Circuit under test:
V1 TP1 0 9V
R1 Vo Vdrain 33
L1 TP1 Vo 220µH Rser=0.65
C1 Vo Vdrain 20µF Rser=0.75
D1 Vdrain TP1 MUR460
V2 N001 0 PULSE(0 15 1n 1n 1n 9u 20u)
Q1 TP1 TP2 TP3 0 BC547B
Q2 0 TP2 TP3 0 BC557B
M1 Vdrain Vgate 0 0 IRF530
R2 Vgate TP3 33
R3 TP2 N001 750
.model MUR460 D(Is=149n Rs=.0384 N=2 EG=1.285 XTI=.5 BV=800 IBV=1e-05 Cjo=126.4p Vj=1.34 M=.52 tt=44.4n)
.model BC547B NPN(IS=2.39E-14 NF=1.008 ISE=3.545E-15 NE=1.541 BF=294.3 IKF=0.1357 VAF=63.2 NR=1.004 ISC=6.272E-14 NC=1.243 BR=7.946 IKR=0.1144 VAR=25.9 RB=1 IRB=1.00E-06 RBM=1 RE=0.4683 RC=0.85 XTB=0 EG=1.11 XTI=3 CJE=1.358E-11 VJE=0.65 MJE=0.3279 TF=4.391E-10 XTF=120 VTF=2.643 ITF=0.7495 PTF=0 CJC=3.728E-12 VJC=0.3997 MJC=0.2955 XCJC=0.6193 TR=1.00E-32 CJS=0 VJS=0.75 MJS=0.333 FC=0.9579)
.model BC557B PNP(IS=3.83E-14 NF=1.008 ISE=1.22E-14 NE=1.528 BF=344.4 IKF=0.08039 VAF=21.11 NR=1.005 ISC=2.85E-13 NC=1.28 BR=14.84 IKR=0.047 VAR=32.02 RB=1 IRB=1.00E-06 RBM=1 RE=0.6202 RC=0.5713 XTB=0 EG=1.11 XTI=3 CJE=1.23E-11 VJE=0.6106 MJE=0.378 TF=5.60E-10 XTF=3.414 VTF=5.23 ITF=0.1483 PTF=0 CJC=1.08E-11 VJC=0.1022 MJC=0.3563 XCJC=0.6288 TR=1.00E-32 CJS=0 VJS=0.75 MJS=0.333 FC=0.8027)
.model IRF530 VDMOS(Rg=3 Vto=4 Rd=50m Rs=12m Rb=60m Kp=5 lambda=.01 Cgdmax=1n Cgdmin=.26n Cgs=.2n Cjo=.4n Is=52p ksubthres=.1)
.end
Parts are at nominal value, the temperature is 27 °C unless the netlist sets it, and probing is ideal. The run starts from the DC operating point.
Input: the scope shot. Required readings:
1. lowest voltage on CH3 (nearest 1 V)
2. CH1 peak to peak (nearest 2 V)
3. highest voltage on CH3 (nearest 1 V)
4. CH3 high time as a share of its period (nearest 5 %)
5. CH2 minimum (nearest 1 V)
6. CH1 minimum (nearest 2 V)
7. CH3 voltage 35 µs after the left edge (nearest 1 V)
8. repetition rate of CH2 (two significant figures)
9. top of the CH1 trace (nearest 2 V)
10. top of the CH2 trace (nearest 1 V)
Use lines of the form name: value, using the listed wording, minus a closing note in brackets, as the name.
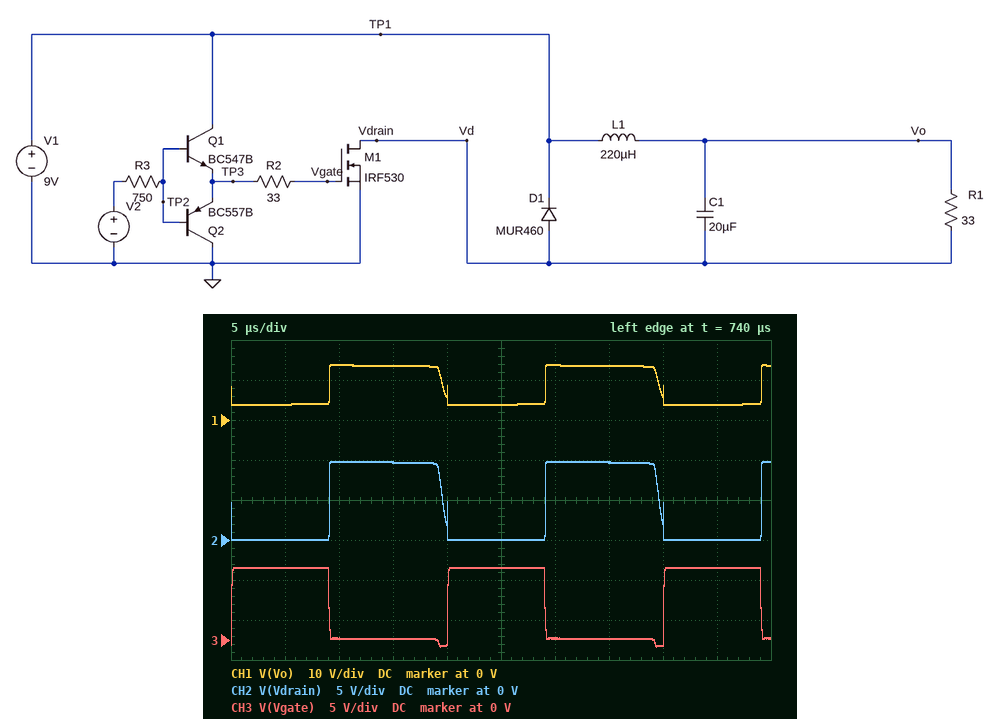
lowest voltage on CH3: -1 V
CH1 peak to peak: 10 V
highest voltage on CH3: 9 V
CH3 high time as a share of its period: 45 %
CH2 minimum: 0 V
CH1 minimum: 4 V
CH3 voltage 35 µs after the left edge: 0 V
repetition rate of CH2: 50 kHz
top of the CH1 trace: 14 V
top of the CH2 trace: 10 V
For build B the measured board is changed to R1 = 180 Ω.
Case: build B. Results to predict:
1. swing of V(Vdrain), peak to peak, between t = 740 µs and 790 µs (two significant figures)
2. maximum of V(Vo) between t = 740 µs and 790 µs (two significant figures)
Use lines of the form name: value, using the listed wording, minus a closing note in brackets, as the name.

swing of V(Vdrain), peak to peak, between t = 740 µs and 790 µs: 10 V
maximum of V(Vo) between t = 740 µs and 790 µs: 16 V
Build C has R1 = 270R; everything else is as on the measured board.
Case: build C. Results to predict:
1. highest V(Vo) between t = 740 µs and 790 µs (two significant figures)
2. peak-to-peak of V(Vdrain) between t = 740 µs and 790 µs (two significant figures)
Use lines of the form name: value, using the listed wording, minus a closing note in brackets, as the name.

highest V(Vo) between t = 740 µs and 790 µs: 16 V
peak-to-peak of V(Vdrain) between t = 740 µs and 790 µs: 10 V
